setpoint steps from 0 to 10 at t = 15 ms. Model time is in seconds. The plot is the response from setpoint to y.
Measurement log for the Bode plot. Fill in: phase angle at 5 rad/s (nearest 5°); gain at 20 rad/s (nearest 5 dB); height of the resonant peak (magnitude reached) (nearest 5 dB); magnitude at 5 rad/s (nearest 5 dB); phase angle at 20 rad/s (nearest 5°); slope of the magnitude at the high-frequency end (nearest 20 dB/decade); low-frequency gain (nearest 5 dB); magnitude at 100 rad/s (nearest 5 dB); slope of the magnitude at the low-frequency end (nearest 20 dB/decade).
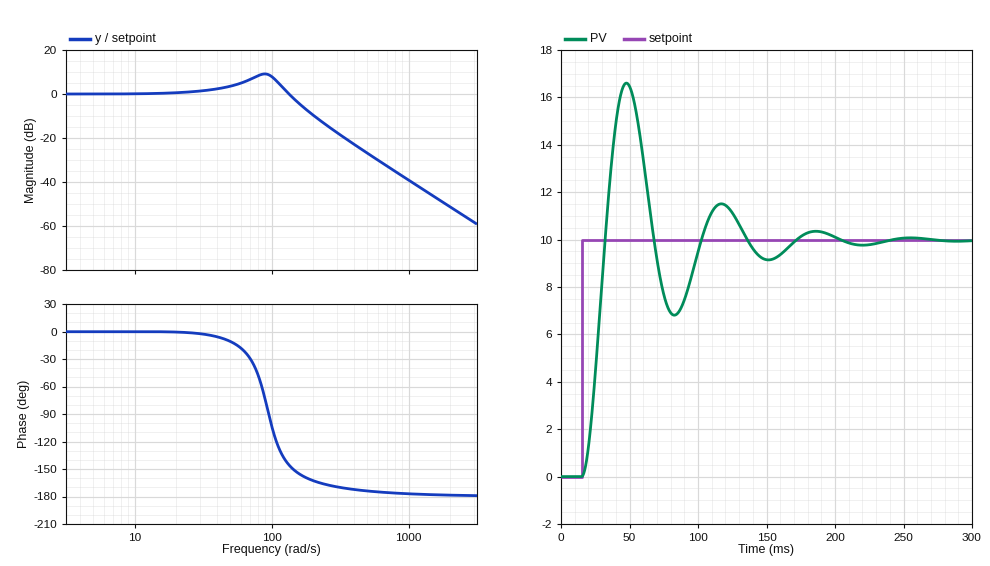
0°
0 dB
10 dB
0 dB
0°
-40 dB/decade
0 dB
10 dB
0 dB/decade
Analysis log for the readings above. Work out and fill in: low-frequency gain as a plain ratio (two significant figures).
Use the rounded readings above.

1.0
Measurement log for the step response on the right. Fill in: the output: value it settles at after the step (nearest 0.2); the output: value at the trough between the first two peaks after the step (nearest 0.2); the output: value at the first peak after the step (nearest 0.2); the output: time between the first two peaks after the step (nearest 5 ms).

10.0
6.8
16.6
70 ms
